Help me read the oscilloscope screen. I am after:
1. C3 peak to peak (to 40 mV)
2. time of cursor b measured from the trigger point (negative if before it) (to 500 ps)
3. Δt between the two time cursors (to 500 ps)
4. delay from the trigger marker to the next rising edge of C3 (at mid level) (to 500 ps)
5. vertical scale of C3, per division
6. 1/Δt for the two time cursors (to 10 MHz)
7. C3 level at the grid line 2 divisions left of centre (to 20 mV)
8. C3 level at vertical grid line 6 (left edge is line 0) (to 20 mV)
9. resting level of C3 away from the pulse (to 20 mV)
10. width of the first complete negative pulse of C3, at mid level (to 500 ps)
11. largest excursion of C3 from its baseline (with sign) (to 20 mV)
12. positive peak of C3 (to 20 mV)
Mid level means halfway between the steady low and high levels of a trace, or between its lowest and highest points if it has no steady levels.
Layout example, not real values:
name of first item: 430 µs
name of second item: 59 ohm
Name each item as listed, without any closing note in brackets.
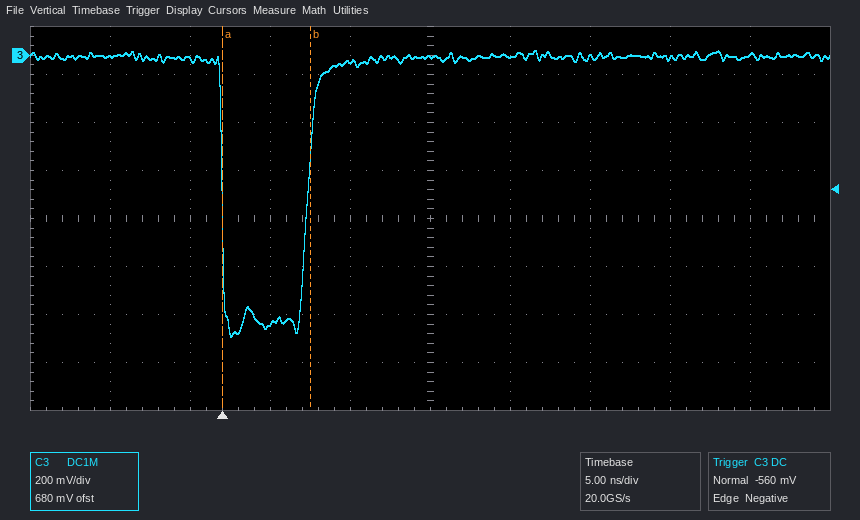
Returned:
C3 peak to peak: 1.20 V
time of cursor b measured from the trigger point (negative if before it): +5.5 ns
Δt between the two time cursors: 5.5 ns
delay from the trigger marker to the next rising edge of C3 (at mid level): 5.5 ns
vertical scale of C3, per division: 200 mV
1/Δt for the two time cursors: 180 MHz
C3 level at the grid line 2 divisions left of centre: -1.12 V
C3 level at vertical grid line 6 (left edge is line 0): 0 mV
resting level of C3 away from the pulse: 0 mV
width of the first complete negative pulse of C3, at mid level: 5.5 ns
largest excursion of C3 from its baseline (with sign): -1.16 V
positive peak of C3: 20 mV
